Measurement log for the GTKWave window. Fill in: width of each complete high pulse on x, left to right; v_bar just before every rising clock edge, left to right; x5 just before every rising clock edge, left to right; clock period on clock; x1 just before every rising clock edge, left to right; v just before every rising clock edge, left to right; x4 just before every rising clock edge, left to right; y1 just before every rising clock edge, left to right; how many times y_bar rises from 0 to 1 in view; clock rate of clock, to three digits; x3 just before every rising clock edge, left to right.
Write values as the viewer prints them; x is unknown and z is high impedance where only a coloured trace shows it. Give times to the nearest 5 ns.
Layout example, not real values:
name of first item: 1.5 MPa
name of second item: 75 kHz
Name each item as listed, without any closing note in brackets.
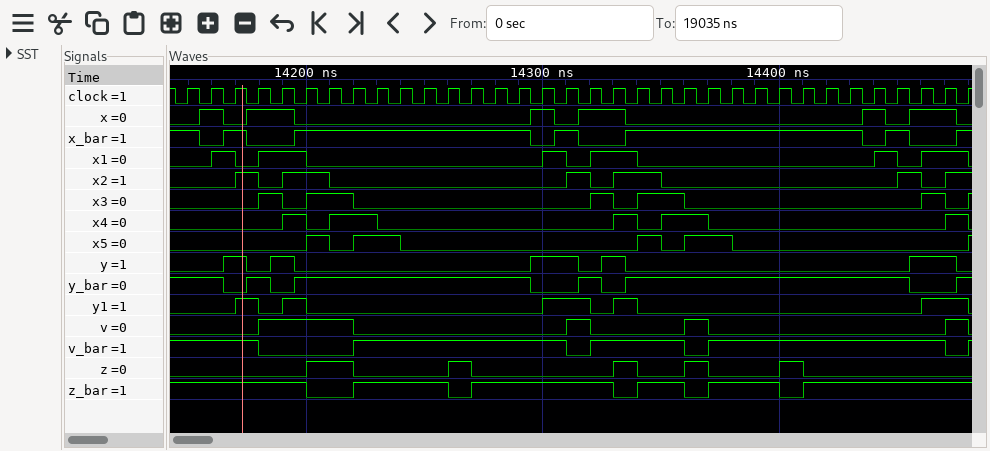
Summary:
width of each complete high pulse on x, left to right: 10 ns, 20 ns, 10 ns, 20 ns, 10 ns, 20 ns
v_bar just before every rising clock edge, left to right: 1 1 1 1 0 0 0 0 1 1 1 1 1 1 1 1 1 0 1 1 1 1 0 1 1 1 1 1 1 1 1 1 1 0
x5 just before every rising clock edge, left to right: 0 0 0 0 0 0 1 0 1 1 0 0 0 0 0 0 0 0 0 0 1 0 1 1 0 0 0 0 0 0 0 0 0 0
clock period on clock: 10 ns
x1 just before every rising clock edge, left to right: 0 0 1 0 1 1 0 0 0 0 0 0 0 0 0 0 1 0 1 1 0 0 0 0 0 0 0 0 0 0 1 0 1 1
v just before every rising clock edge, left to right: 0 0 0 0 1 1 1 1 0 0 0 0 0 0 0 0 0 1 0 0 0 0 1 0 0 0 0 0 0 0 0 0 0 1
x4 just before every rising clock edge, left to right: 0 0 0 0 0 1 0 1 1 0 0 0 0 0 0 0 0 0 0 1 0 1 1 0 0 0 0 0 0 0 0 0 0 1
y1 just before every rising clock edge, left to right: 0 0 0 1 0 1 0 0 0 0 0 0 0 0 0 0 1 1 0 1 0 0 0 0 0 0 0 0 0 0 0 0 1 1
how many times y_bar rises from 0 to 1 in view: 5
clock rate of clock, to three digits: 100 MHz
x3 just before every rising clock edge, left to right: 0 0 0 0 1 0 1 1 0 0 0 0 0 0 0 0 0 0 1 0 1 1 0 0 0 0 0 0 0 0 0 0 1 0
